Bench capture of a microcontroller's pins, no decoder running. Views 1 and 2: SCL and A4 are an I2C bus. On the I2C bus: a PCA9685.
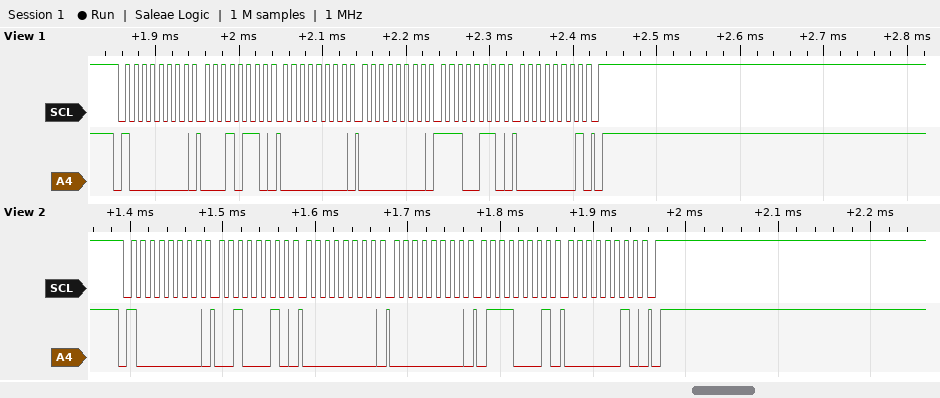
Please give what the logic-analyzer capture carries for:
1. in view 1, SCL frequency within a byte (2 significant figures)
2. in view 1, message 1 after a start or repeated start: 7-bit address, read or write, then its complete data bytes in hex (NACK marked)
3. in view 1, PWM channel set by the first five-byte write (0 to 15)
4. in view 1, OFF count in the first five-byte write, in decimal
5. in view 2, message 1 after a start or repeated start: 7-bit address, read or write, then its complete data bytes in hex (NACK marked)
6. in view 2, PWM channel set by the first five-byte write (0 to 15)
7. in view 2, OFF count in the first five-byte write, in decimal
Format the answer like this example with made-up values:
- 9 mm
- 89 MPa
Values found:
- 100 kHz
- 0x40 write: 16 00 00 E6 01
- 4
- 486
- 0x40 write: 22 00 00 71 02
- 7
- 625
